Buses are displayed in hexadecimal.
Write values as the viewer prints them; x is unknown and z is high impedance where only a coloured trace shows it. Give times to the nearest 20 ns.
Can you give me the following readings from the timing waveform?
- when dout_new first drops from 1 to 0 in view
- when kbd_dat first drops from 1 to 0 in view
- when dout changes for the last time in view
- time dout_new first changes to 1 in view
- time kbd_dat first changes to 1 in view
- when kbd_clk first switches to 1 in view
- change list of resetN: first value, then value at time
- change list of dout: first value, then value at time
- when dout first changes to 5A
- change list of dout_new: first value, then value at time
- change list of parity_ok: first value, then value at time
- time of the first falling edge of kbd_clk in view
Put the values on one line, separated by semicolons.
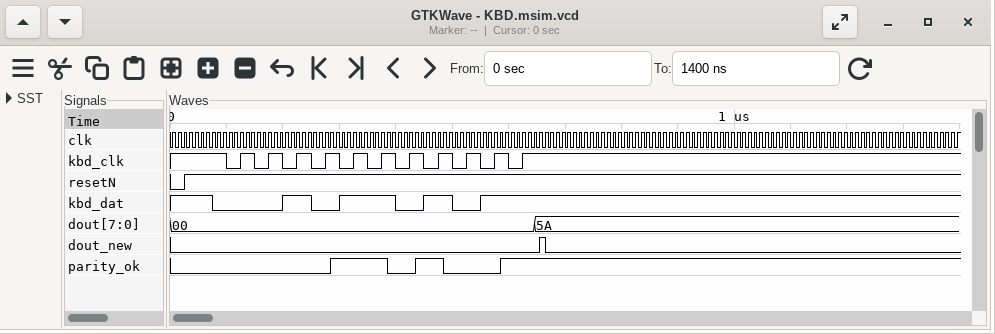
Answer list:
660 ns; 80 ns; 640 ns; 660 ns; 200 ns; 120 ns; 0, 1 at 20 ns; 00, 5A at 640 ns; 640 ns; 0, 1 at 660 ns, 0 at 660 ns; 0, 1 at 280 ns, 0 at 380 ns, 1 at 440 ns, 0 at 480 ns, 1 at 580 ns; 100 ns
